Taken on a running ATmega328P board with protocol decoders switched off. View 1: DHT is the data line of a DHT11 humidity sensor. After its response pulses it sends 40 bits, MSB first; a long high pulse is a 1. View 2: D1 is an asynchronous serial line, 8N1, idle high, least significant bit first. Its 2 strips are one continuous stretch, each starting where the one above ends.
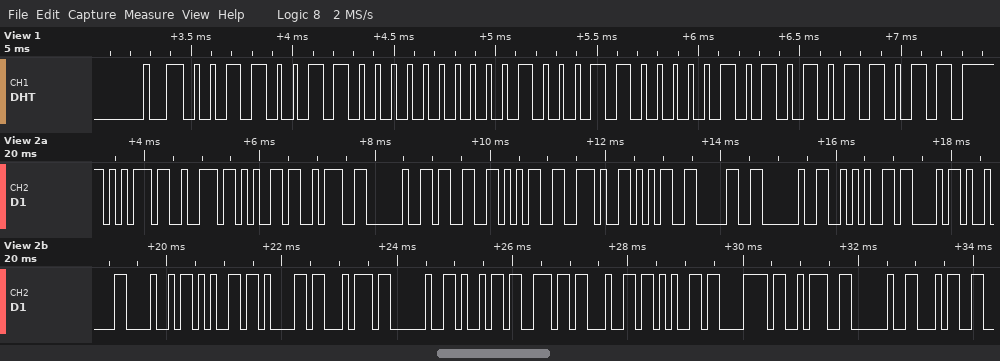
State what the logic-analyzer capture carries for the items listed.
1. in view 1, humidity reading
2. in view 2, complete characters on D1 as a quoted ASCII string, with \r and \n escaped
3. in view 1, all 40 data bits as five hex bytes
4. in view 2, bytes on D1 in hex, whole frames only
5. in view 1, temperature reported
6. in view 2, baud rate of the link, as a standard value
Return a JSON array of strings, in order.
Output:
["51 %", "\"ure: 35.50 *C\\tHeat index: 4\"", "33 00 23 05 5B", "75 72 65 3A 20 33 35 2E 35 30 20 2A 43 09 48 65 61 74 20 69 6E 64 65 78 3A 20 34", "35.5 °C", "9600 baud"]
